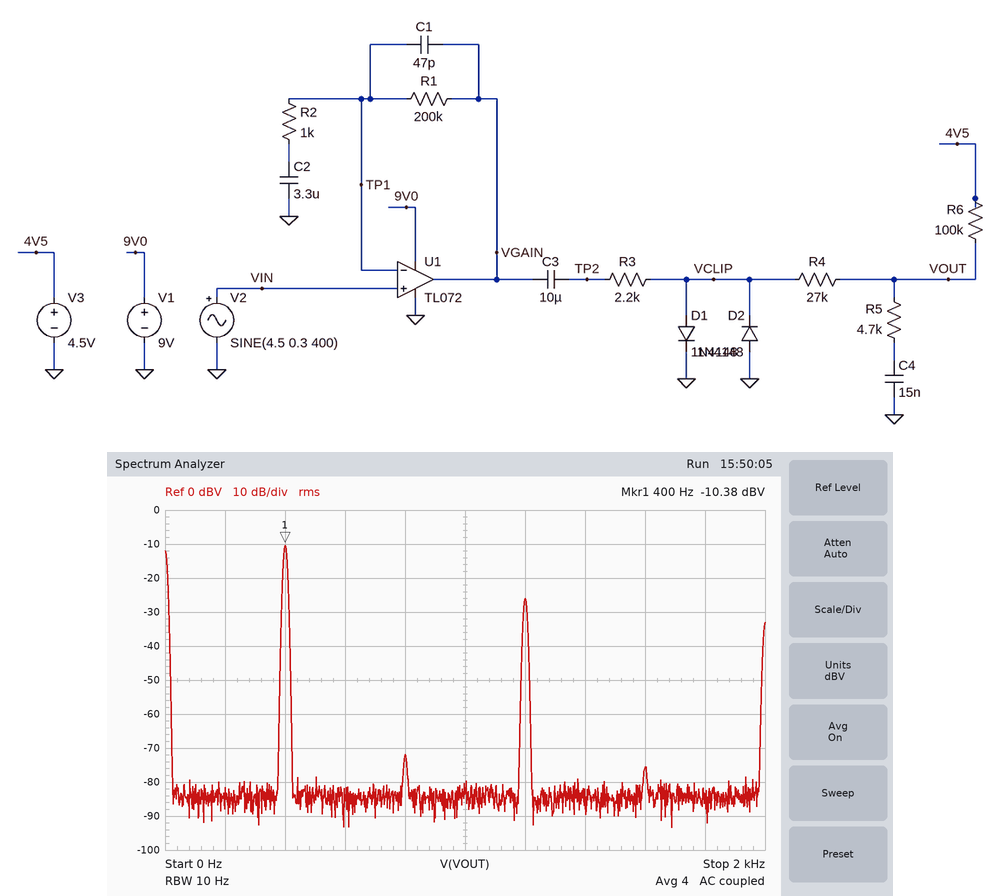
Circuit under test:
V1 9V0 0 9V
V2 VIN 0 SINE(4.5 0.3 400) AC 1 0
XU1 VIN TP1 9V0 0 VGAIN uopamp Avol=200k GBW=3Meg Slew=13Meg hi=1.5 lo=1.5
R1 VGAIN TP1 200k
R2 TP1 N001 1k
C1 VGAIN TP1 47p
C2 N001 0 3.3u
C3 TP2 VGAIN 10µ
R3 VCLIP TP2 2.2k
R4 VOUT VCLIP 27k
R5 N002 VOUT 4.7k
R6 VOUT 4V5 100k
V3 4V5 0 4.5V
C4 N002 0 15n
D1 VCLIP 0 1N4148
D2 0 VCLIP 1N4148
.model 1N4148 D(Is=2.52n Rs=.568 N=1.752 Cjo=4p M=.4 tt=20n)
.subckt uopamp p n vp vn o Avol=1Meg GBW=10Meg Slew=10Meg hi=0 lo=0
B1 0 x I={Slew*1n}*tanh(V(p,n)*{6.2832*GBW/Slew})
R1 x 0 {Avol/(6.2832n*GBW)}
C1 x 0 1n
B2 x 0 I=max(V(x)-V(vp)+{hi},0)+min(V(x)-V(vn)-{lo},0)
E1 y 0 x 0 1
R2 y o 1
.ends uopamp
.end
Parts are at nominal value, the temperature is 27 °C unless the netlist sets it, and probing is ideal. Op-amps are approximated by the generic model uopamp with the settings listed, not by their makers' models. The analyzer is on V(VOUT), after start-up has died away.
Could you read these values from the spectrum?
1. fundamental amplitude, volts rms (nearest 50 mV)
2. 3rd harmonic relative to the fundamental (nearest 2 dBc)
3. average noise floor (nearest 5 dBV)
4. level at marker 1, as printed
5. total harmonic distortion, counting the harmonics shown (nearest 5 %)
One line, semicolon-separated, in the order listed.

300 mV; -16 dBc; -85 dBV; -10.38 dBV; 15 %
